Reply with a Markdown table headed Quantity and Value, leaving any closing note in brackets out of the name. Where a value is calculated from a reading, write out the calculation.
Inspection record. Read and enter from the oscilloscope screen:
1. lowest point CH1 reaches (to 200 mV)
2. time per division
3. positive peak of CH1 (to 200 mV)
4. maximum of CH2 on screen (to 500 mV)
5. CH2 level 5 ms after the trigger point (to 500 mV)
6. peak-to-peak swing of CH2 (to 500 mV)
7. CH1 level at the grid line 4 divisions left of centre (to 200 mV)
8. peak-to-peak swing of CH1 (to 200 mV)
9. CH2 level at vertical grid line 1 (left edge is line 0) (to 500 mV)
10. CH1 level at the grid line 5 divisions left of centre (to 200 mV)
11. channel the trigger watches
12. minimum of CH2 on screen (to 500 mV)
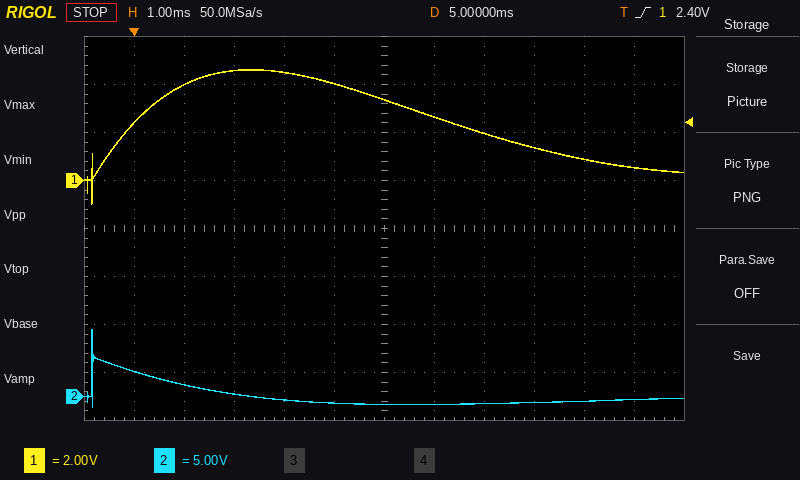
| Quantity | Value |
|---|---|
| lowest point CH1 reaches | -1.0 V |
| time per division | 1 ms |
| positive peak of CH1 | 4.6 V |
| maximum of CH2 on screen | 7.0 V |
| CH2 level 5 ms after the trigger point | -1.0 V |
| peak-to-peak swing of CH2 | 7.0 V − (-1.0 V) = 8.0 V |
| CH1 level at the grid line 4 divisions left of centre | 4.0 V |
| peak-to-peak swing of CH1 | 4.6 V − (-1.0 V) = 5.6 V |
| CH2 level at vertical grid line 1 (left edge is line 0) | 2.5 V |
| CH1 level at the grid line 5 divisions left of centre | 2.4 V |
| channel the trigger watches | CH1 |
| minimum of CH2 on screen | -1.0 V |
